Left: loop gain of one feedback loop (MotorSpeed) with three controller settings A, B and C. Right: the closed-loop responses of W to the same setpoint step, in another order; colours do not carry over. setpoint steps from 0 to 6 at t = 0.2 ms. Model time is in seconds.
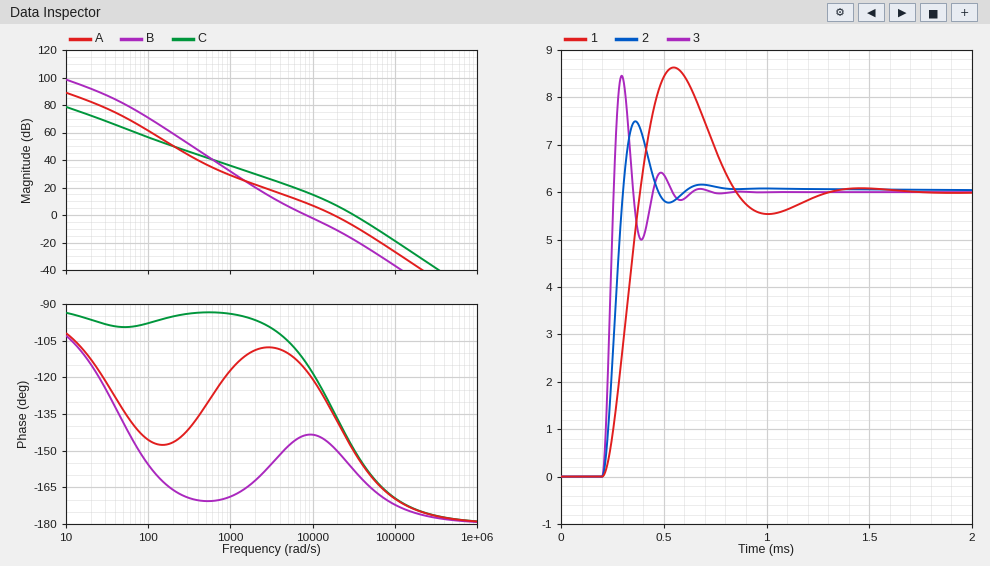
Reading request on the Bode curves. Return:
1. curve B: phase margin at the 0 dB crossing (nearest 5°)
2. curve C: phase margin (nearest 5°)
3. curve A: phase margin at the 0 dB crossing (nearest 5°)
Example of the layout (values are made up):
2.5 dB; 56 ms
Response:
35°; 30°; 45°
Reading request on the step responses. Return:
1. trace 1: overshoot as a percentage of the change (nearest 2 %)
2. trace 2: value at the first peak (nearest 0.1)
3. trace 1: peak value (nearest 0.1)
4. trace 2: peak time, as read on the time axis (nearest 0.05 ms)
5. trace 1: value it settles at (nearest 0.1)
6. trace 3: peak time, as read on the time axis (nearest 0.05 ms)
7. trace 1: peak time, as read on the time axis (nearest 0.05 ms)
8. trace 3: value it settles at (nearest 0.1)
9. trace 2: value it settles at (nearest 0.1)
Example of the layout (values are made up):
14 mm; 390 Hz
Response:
44 %; 7.5; 8.6; 0.35 ms; 6.0; 0.30 ms; 0.55 ms; 6.0; 6.0
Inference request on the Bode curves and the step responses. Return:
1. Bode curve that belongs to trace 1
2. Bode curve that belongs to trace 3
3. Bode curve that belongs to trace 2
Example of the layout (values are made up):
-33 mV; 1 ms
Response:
B; C; A
